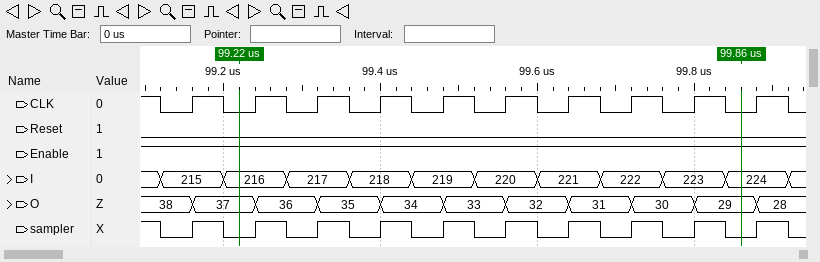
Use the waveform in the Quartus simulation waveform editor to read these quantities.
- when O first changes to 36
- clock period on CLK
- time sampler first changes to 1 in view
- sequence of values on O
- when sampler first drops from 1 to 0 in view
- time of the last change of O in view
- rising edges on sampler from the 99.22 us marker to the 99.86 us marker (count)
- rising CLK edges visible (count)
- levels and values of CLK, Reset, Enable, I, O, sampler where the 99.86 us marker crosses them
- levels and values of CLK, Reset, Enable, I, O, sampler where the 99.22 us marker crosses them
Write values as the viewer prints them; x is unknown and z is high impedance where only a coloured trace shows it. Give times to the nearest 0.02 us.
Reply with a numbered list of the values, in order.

1. 99.24 us
2. 0.08 us
3. 99.16 us
4. 38, 37, 36, 35, 34, 33, 32, 31, 30, 29, 28
5. 99.12 us
6. 99.88 us
7. 8
8. 10
9. CLK=0, Reset=0, Enable=1, I=224, O=29, sampler=0
10. CLK=0, Reset=0, Enable=1, I=216, O=37, sampler=0
